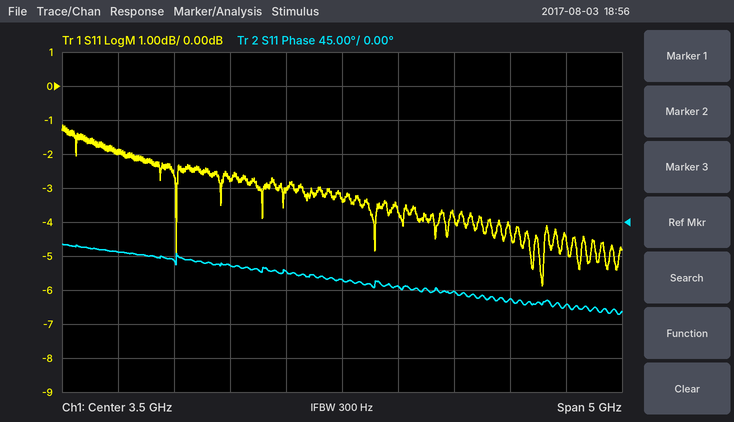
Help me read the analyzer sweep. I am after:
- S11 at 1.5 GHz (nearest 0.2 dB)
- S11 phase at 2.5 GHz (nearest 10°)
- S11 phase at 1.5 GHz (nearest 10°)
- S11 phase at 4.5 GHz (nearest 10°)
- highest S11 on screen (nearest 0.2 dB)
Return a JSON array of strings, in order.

["-2.0 dB", "-60°", "-40°", "-90°", "-1.2 dB"]
